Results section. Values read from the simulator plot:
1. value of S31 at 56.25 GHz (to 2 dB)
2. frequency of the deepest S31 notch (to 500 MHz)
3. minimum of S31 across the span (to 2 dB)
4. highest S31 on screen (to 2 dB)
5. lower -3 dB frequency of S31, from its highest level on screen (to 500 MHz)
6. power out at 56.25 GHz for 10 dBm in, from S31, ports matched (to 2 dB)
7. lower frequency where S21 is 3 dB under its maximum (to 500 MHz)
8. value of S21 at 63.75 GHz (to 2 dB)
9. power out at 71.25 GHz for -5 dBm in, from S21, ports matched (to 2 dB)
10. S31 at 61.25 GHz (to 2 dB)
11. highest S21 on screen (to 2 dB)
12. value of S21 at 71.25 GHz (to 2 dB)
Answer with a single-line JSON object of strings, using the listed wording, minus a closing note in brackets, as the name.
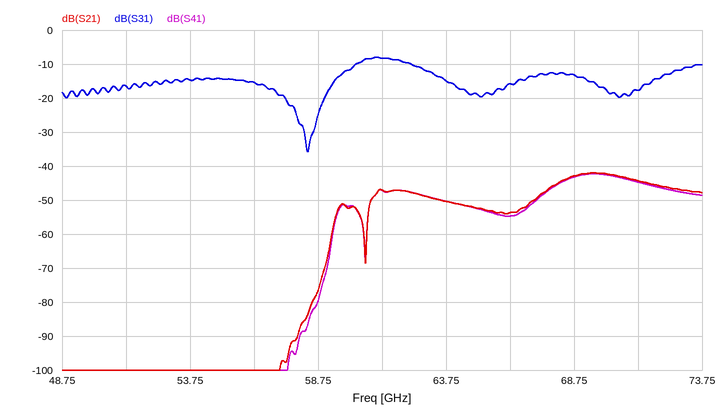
{"value of S31 at 56.25 GHz": "-16 dB", "frequency of the deepest S31 notch": "58.5 GHz", "minimum of S31 across the span": "-36 dB", "highest S31 on screen": "-8 dB", "lower -3 dB frequency of S31, from its highest level on screen": "60.0 GHz", "power out at 56.25 GHz for 10 dBm in, from S31, ports matched": "-6 dBm", "lower frequency where S21 is 3 dB under its maximum": "68.0 GHz", "value of S21 at 63.75 GHz": "-50 dB", "power out at 71.25 GHz for -5 dBm in, from S21, ports matched": "-50 dBm", "S31 at 61.25 GHz": "-8 dB", "highest S21 on screen": "-42 dB", "value of S21 at 71.25 GHz": "-44 dB"}
